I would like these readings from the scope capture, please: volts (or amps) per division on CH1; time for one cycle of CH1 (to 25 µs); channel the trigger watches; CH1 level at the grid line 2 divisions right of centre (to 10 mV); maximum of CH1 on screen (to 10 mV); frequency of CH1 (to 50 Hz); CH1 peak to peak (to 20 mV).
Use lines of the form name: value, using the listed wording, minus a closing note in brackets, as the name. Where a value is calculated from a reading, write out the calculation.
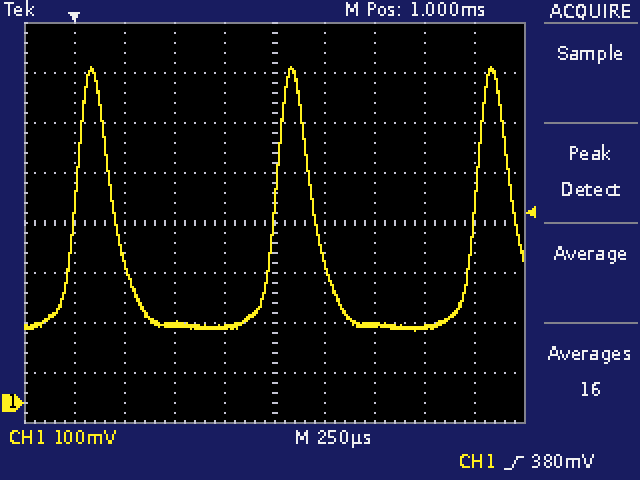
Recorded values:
volts (or amps) per division on CH1: 100 mV
time for one cycle of CH1: 1.000 ms
channel the trigger watches: CH1
CH1 level at the grid line 2 divisions right of centre: 160 mV
maximum of CH1 on screen: 670 mV
frequency of CH1: 1 / 1.000 ms ≈ 1.00 kHz
CH1 peak to peak: 520 mV
